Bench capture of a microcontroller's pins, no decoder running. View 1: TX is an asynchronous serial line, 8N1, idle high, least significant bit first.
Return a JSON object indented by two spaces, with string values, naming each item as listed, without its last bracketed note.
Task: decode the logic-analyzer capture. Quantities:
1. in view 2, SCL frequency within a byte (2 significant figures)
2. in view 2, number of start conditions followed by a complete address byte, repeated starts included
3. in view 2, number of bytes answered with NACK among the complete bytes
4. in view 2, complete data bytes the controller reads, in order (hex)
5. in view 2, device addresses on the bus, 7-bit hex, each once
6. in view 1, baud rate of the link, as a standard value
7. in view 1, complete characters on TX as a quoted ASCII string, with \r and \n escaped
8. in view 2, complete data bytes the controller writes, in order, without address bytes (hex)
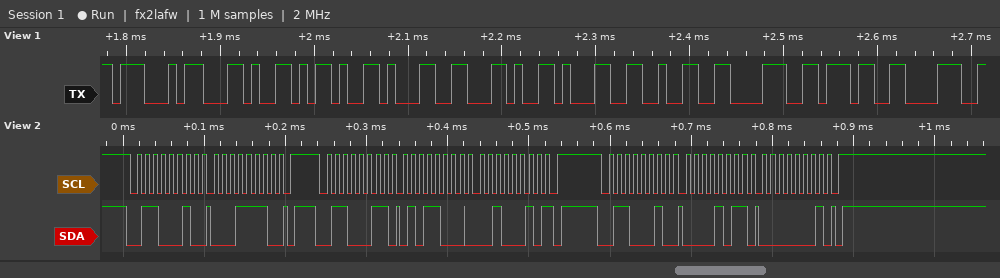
{
  "in view 2, SCL frequency within a byte": "100 kHz",
  "in view 2, number of start conditions followed by a complete address byte, repeated starts included": "3",
  "in view 2, number of bytes answered with NACK among the complete bytes": "1",
  "in view 2, complete data bytes the controller reads, in order": "58 22",
  "in view 2, device addresses on the bus, 7-bit hex, each once": "0x31",
  "in view 1, baud rate of the link, as a standard value": "115200 baud",
  "in view 1, complete characters on TX as a quoted ASCII string, with \\r and \\n escaped": "\"G,-1,12878\"",
  "in view 2, complete data bytes the controller writes, in order, without address bytes": "1E 0B 01"
}
